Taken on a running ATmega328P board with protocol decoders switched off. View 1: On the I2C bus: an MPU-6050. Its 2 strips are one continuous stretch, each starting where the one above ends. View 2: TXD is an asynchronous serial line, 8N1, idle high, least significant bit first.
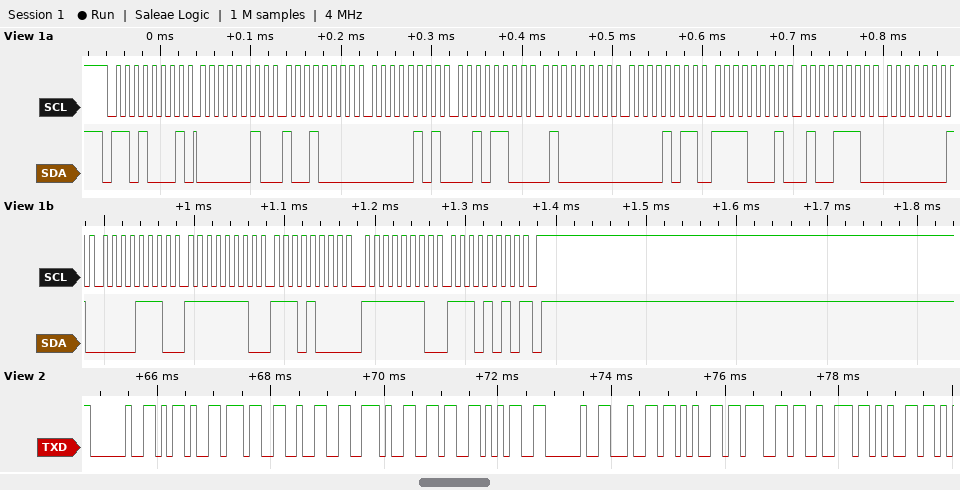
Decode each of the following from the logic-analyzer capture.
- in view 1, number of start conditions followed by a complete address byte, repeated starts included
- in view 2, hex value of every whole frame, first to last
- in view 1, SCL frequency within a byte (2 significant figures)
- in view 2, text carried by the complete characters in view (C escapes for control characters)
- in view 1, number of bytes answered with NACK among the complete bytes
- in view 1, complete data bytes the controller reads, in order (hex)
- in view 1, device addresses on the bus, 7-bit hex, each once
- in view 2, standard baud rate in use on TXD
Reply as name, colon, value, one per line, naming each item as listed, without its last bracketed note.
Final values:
in view 1, number of start conditions followed by a complete address byte, repeated starts included: 1
in view 2, hex value of every whole frame, first to last: 20 2D 37 32 2E 36 35 20 64 65 67 72 65
in view 1, SCL frequency within a byte: 100 kHz
in view 2, text carried by the complete characters in view: " -72.65 degre"
in view 1, number of bytes answered with NACK among the complete bytes: 1
in view 1, complete data bytes the controller reads, in order: 02 90 05 2C 40 0B F1 4E 01 0E FE E8 FE EA
in view 1, device addresses on the bus, 7-bit hex, each once: 0x68
in view 2, standard baud rate in use on TXD: 9600 baud
